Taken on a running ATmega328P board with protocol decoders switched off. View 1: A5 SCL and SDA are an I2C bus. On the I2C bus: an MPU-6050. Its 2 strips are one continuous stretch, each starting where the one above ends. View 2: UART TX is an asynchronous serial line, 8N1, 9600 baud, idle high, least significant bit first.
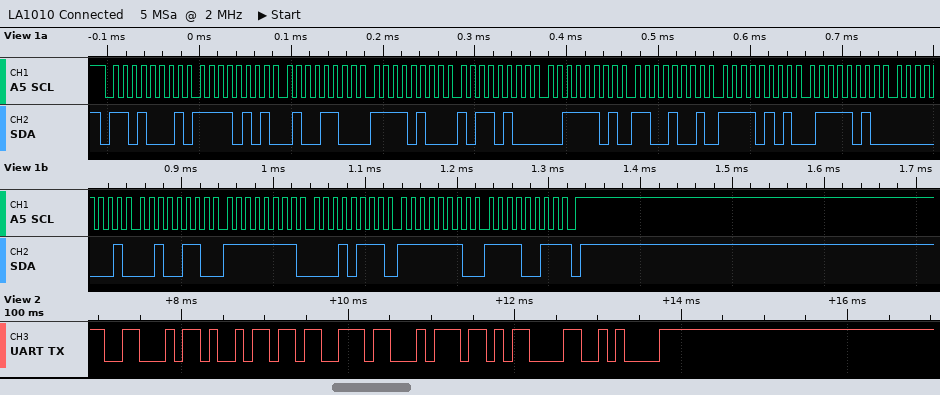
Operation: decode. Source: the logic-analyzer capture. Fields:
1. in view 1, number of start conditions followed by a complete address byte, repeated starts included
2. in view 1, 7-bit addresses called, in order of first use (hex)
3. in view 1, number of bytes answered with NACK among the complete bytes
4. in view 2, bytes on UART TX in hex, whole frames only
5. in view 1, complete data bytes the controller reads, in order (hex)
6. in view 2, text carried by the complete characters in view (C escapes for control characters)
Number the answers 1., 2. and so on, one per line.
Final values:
1. 1
2. 0x68
3. 1
4. 0x46 0x69 0x73 0x74 0x0D 0x0A
5. F5 4C F4 B4 3D C9 F5 7A 01 26 FF 17 FE F3
6. "Fist\r\n"
